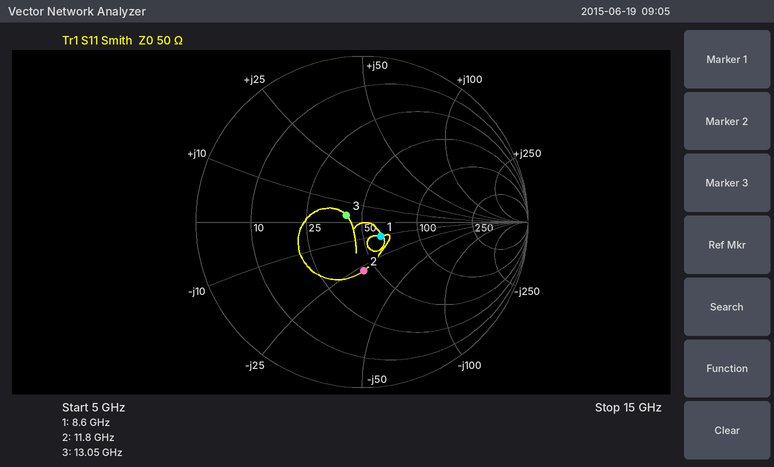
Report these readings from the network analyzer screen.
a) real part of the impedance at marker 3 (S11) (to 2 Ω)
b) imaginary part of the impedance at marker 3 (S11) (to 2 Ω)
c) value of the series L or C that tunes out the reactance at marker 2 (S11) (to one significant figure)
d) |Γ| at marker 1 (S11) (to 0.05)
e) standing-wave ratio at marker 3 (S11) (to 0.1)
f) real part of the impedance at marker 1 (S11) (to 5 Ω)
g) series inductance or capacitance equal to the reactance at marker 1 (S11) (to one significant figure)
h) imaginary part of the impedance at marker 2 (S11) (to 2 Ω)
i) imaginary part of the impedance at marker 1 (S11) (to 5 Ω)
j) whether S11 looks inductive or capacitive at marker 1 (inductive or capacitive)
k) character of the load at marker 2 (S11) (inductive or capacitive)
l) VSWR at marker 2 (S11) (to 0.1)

42 Ω
+4 Ω
400 pH
0.15
1.2
60 Ω
2 pF
-28 Ω
-10 Ω
capacitive
capacitive
1.8
